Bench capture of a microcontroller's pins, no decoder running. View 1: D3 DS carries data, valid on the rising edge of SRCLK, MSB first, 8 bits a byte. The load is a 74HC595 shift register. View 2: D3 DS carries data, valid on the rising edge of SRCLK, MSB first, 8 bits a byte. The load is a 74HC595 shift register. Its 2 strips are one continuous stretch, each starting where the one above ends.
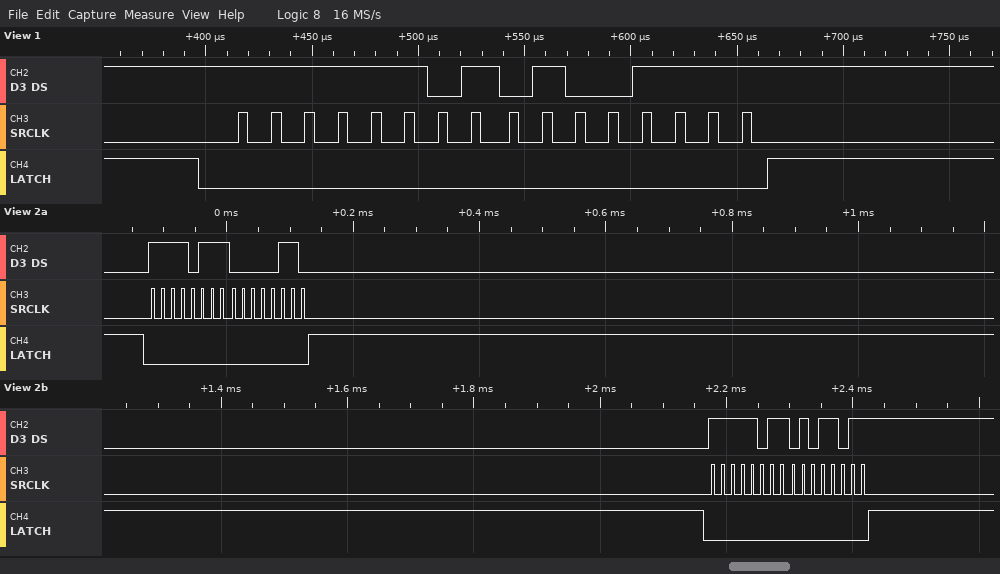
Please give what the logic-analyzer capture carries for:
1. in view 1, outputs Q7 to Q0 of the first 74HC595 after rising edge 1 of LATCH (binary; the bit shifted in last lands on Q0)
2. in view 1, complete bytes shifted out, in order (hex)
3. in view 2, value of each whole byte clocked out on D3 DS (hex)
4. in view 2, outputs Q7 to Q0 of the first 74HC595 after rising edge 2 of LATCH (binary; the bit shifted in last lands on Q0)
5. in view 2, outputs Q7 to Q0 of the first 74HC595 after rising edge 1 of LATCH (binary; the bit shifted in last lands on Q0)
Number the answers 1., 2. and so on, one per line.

1. 01001111
2. 0xFD 0x4F
3. 0xF7 0x06 0xFB 0x5B
4. 01011011
5. 00000110
